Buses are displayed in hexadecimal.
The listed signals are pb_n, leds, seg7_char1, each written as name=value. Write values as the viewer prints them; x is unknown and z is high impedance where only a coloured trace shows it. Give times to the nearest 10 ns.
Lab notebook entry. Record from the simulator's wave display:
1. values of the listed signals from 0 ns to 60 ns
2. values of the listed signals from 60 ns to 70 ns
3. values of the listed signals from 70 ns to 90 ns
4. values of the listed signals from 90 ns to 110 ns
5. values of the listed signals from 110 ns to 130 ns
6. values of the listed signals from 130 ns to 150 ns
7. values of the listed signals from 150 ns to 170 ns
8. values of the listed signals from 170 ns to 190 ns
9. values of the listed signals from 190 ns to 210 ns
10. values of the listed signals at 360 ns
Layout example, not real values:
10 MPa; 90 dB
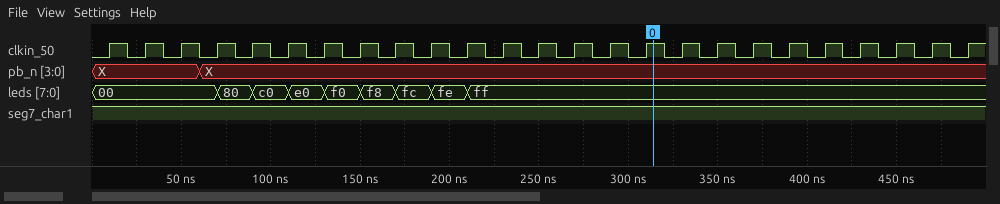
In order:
pb_n=X, leds=00, seg7_char1=1; pb_n=X, leds=00, seg7_char1=1; pb_n=X, leds=80, seg7_char1=1; pb_n=X, leds=c0, seg7_char1=1; pb_n=X, leds=e0, seg7_char1=1; pb_n=X, leds=f0, seg7_char1=1; pb_n=X, leds=f8, seg7_char1=1; pb_n=X, leds=fc, seg7_char1=1; pb_n=X, leds=fe, seg7_char1=1; pb_n=X, leds=ff, seg7_char1=1
